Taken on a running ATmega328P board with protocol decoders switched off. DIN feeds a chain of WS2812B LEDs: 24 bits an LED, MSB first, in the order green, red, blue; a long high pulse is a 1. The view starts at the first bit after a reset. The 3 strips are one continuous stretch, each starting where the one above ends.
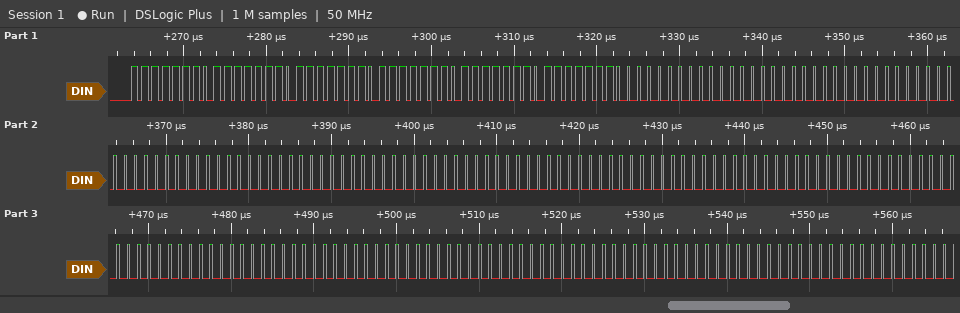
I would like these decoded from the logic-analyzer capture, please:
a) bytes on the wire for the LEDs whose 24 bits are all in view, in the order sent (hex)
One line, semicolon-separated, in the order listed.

FE FE FE FE FE FE 00 00 00 00 00 00 00 00 00 00 00 00 00 00 00 00 00 00 00 00 00 00 00 00
